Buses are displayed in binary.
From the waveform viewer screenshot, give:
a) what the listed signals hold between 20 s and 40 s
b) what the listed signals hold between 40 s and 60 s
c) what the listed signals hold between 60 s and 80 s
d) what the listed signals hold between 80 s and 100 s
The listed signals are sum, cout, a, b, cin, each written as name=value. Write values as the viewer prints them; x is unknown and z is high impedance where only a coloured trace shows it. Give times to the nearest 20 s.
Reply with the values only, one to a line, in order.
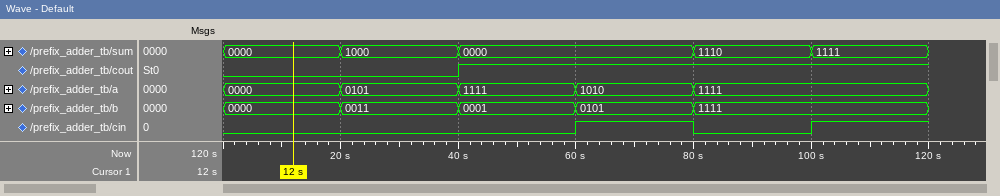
sum=1000, cout=0, a=0101, b=0011, cin=0
sum=0000, cout=1, a=1111, b=0001, cin=0
sum=0000, cout=1, a=1010, b=0101, cin=1
sum=1110, cout=1, a=1111, b=1111, cin=0
